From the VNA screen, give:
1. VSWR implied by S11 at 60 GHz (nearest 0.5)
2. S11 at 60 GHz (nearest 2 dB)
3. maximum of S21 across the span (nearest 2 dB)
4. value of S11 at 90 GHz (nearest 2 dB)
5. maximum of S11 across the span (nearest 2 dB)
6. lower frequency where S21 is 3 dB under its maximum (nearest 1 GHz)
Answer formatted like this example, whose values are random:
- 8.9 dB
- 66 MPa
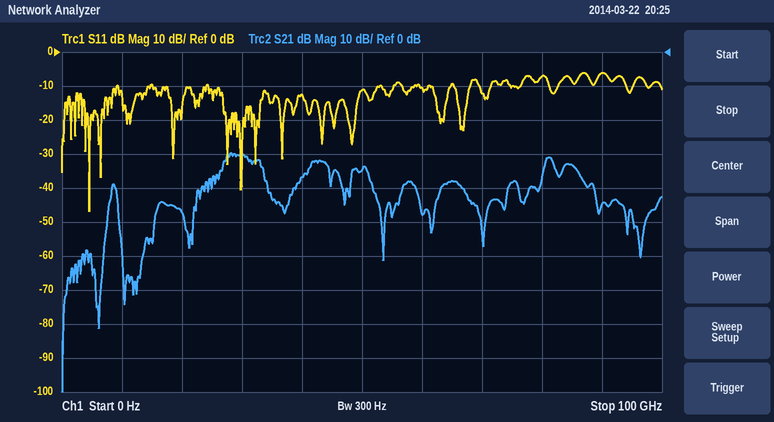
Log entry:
- 2.0
- -10 dB
- -30 dB
- -6 dB
- -6 dB
- 27 GHz
